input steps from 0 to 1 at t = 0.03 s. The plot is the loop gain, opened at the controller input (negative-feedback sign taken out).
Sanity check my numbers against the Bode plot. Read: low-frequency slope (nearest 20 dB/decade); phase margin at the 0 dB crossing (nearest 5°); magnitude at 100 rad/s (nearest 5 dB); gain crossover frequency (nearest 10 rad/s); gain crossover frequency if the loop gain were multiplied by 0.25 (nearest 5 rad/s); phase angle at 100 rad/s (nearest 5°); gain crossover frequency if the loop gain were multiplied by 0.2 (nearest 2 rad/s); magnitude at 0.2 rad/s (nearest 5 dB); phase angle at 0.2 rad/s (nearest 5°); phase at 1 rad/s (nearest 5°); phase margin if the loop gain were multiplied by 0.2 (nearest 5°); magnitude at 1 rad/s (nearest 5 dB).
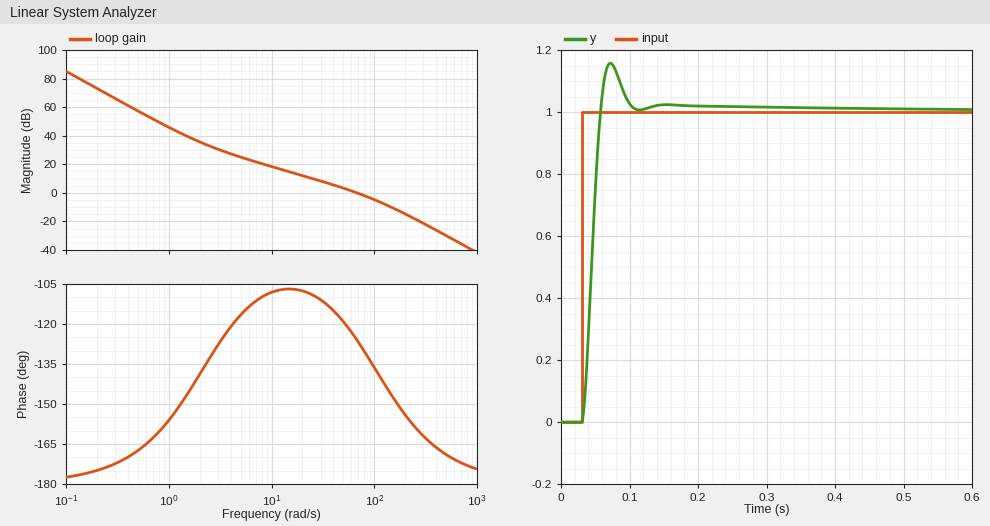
-40 dB/decade
55°
-5 dB
70 rad/s
20 rad/s
-135°
16 rad/s
75 dB
-175°
-155°
75°
45 dB
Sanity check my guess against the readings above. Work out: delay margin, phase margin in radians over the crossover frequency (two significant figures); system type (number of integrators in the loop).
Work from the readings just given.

0.014 s
2
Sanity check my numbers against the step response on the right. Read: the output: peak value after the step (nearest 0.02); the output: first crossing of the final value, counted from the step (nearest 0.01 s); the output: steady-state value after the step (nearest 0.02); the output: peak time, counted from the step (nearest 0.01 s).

1.16
0.03 s
1.00
0.04 s
